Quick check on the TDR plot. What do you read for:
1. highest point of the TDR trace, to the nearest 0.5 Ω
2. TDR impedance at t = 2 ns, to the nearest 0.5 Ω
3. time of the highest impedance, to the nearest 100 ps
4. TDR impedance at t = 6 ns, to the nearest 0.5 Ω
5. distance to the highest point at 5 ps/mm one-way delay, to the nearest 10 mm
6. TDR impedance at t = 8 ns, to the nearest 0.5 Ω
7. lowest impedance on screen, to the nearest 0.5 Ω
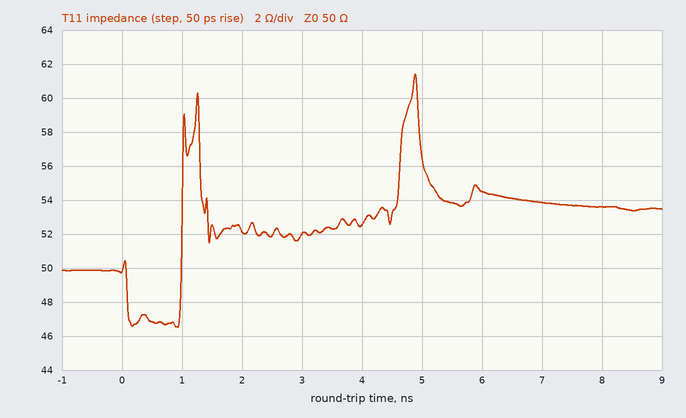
61.5 Ω
52.0 Ω
4.9 ns
54.5 Ω
490 mm
53.5 Ω
46.5 Ω
